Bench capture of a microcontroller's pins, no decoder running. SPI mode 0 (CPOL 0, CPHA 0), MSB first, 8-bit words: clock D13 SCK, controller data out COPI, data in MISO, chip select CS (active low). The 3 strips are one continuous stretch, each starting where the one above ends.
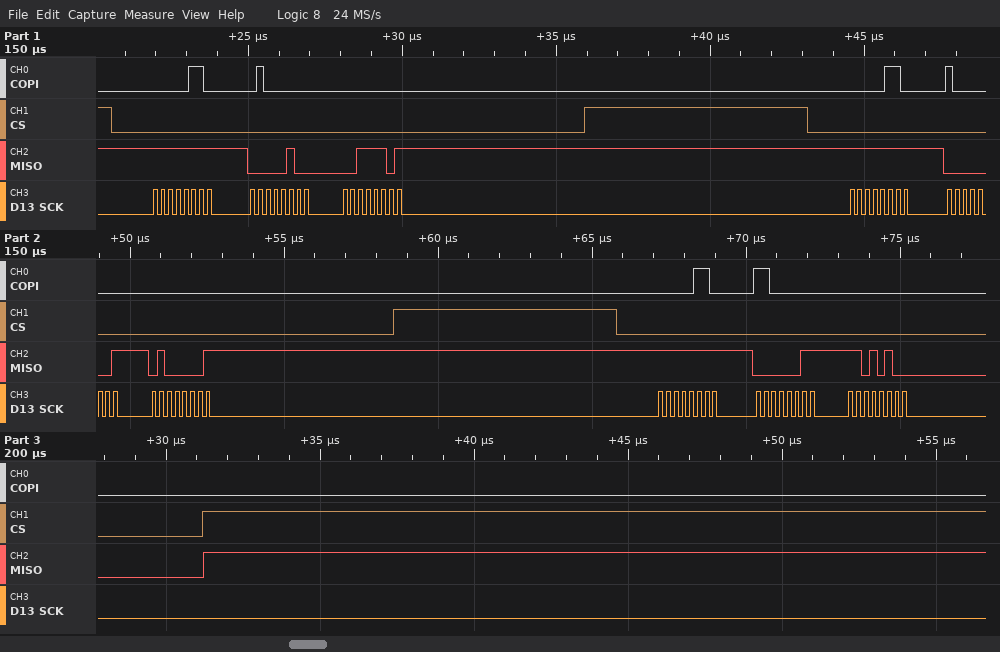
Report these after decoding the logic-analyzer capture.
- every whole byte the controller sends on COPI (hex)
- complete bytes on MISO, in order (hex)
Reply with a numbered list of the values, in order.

1. 06 40 00 06 80 00 06 C0 00
2. FF 04 3D FF 01 41 FF 03 D4
